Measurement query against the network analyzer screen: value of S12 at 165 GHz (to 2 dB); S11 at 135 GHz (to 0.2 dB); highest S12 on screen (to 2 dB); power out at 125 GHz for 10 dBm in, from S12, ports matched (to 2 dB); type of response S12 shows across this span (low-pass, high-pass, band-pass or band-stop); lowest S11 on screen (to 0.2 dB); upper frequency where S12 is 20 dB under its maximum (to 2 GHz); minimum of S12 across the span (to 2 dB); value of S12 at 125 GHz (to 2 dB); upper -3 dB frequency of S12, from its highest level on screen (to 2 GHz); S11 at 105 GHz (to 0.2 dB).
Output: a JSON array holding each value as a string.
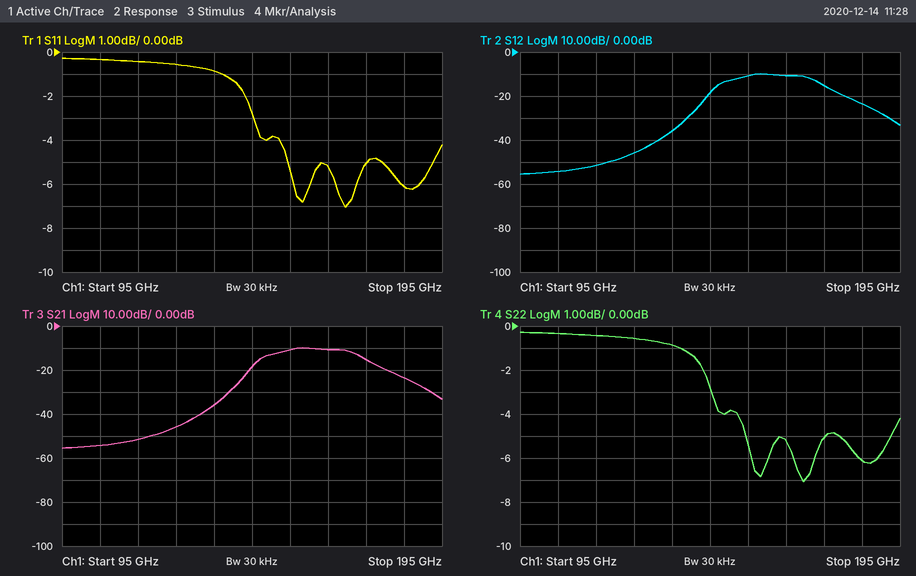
["-10 dB", "-0.8 dB", "-10 dB", "-36 dBm", "band-pass", "-7.0 dB", "192 GHz", "-56 dB", "-46 dB", "172 GHz", "-0.4 dB"]
